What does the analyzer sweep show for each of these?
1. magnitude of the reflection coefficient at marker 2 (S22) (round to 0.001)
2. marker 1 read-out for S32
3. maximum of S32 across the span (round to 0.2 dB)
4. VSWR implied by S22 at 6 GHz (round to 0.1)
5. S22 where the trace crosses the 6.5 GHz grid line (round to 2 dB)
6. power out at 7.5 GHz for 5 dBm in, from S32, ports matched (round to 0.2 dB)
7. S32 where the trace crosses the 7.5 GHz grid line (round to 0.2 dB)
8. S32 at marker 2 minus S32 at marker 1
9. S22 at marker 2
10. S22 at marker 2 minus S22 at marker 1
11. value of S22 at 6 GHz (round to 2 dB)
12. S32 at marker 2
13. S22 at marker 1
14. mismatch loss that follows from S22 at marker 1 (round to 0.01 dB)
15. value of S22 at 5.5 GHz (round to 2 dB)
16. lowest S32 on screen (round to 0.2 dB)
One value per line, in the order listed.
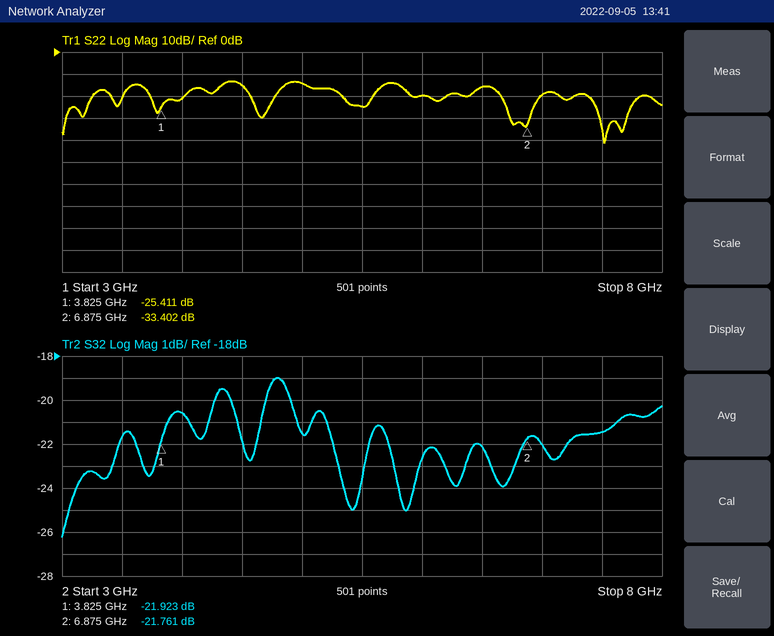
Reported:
0.021
-21.923 dB
-19.0 dB
1.2
-16 dB
-16.4 dBm
-21.4 dB
0.162 dB
-33.402 dB
-7.991 dB
-20 dB
-21.761 dB
-25.411 dB
0.01 dB
-24 dB
-26.2 dB
